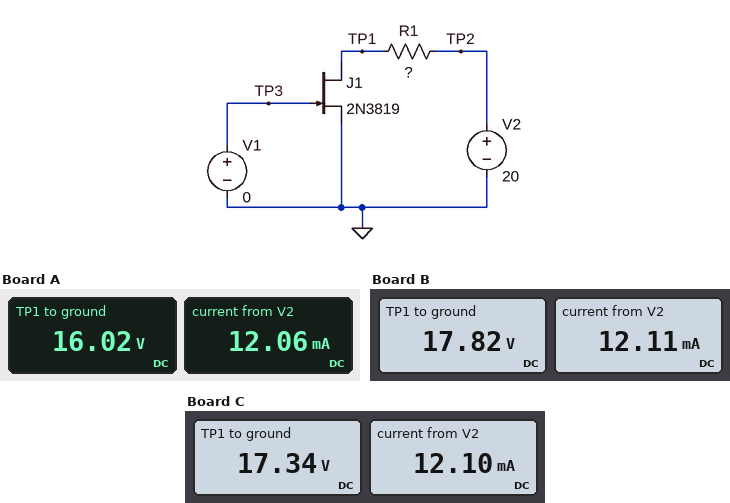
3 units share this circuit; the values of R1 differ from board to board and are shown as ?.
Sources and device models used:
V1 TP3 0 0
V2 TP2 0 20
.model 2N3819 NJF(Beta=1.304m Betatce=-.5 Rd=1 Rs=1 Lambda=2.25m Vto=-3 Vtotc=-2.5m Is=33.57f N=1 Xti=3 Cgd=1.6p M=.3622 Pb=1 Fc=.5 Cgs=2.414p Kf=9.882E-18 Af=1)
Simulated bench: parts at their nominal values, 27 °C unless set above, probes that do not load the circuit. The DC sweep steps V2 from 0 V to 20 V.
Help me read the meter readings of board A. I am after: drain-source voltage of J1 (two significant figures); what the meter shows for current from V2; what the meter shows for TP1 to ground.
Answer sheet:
16 V
12.06 mA
16.02 V
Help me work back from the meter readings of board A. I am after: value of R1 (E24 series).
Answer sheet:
330 Ω
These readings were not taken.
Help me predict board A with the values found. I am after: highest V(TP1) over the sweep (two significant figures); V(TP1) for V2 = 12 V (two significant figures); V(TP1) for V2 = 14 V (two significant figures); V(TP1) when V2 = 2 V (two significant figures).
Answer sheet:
16 V
8.1 V
10 V
610 mV
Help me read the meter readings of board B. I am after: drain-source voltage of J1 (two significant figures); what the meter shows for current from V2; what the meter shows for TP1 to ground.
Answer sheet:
18 V
12.11 mA
17.82 V
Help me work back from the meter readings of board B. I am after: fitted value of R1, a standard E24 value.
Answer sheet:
180 Ω
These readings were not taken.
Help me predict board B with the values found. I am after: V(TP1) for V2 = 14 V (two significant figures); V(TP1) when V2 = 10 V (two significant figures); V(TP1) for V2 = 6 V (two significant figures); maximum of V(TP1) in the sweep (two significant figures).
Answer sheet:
12 V
7.9 V
3.9 V
18 V
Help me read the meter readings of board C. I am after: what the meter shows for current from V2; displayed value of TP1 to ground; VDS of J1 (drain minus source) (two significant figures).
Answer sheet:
12.10 mA
17.34 V
17 V
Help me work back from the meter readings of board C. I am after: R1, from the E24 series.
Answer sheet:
220 Ω
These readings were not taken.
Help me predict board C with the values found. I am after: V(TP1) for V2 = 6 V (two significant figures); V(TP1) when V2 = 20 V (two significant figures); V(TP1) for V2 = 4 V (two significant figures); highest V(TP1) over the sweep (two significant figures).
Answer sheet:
3.4 V
17 V
1.8 V
17 V
